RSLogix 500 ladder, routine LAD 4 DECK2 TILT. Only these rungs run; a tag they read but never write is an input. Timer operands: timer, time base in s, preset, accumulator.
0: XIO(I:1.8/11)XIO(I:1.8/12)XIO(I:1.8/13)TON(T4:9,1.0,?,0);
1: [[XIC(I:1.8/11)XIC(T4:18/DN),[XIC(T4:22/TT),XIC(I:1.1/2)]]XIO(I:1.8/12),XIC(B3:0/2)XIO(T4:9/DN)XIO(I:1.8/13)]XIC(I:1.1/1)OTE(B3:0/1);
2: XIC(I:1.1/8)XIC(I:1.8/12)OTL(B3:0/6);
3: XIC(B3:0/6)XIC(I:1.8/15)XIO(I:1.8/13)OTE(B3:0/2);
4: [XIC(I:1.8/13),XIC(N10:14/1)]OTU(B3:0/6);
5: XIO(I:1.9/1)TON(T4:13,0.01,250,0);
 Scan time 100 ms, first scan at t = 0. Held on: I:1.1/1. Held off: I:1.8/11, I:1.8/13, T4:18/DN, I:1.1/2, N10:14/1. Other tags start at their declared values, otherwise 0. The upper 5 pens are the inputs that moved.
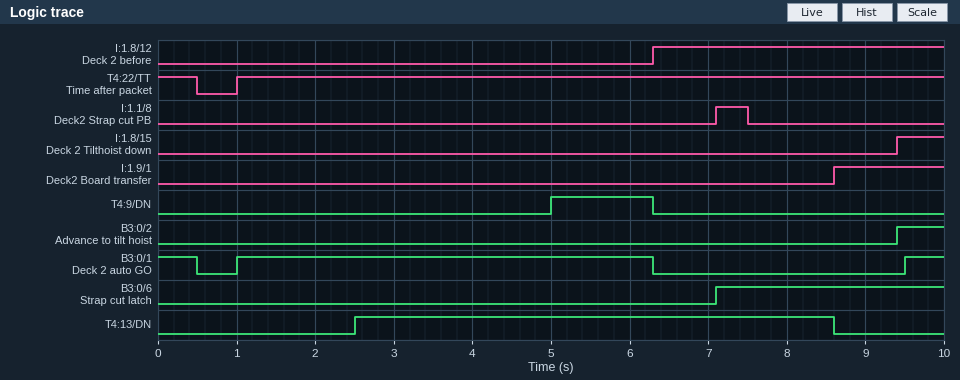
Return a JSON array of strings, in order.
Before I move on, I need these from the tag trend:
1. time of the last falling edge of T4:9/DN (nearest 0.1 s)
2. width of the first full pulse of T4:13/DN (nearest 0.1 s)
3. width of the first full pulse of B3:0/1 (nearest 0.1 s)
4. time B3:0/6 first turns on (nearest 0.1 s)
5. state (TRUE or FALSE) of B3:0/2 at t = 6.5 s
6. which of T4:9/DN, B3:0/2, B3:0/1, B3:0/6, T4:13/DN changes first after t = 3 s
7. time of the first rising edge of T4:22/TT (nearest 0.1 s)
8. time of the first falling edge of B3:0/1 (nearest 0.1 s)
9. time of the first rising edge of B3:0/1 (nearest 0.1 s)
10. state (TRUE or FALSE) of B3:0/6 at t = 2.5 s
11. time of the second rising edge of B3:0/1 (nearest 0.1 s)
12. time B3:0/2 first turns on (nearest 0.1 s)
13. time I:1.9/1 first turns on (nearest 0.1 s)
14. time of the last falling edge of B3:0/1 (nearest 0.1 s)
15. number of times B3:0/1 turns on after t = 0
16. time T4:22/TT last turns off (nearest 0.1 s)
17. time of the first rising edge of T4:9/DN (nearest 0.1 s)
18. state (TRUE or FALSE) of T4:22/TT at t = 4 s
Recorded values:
["6.3 s", "6.1 s", "5.3 s", "7.1 s", "FALSE", "T4:9/DN", "1.0 s", "0.5 s", "1.0 s", "FALSE", "9.5 s", "9.4 s", "8.6 s", "6.3 s", "2", "0.5 s", "5.0 s", "TRUE"]
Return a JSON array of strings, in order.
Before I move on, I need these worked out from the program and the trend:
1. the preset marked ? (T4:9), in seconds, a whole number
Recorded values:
["5 s"]
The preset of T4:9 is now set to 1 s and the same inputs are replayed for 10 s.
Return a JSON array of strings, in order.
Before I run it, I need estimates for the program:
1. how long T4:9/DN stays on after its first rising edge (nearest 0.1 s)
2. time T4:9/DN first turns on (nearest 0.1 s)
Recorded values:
["5.3 s", "1.0 s"]
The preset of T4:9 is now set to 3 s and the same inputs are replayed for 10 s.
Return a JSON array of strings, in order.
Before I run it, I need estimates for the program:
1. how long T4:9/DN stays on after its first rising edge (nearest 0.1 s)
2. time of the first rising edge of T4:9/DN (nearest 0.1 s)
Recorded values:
["3.3 s", "3.0 s"]
